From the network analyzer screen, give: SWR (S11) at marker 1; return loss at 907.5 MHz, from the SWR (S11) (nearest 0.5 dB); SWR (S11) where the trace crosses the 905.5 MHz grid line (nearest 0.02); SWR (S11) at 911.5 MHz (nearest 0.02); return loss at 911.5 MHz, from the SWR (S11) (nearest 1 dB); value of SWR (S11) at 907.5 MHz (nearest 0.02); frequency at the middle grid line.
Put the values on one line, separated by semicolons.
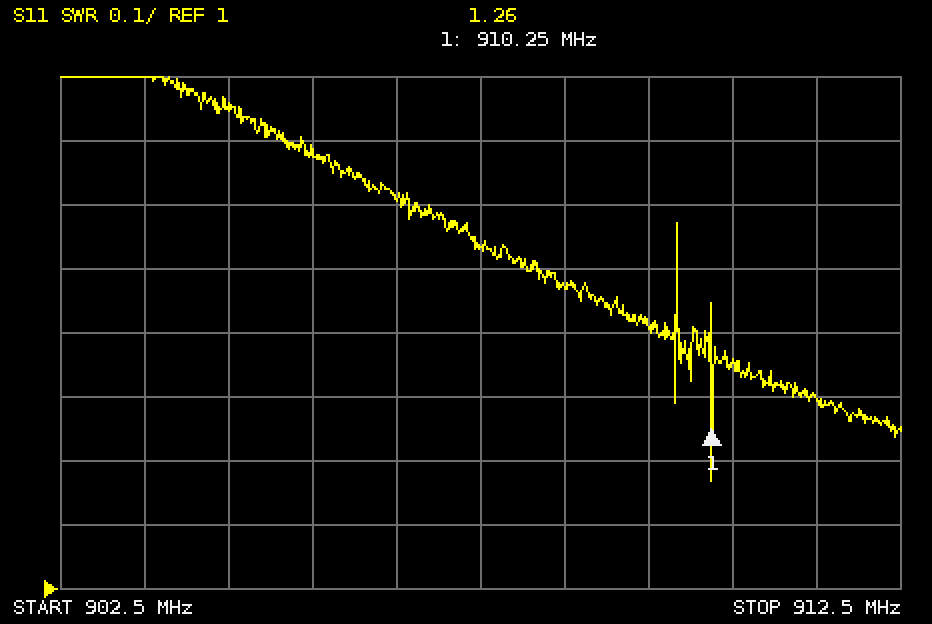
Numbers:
1.26; 13.5 dB; 1.68; 1.30; 18 dB; 1.54; 907.5 MHz
